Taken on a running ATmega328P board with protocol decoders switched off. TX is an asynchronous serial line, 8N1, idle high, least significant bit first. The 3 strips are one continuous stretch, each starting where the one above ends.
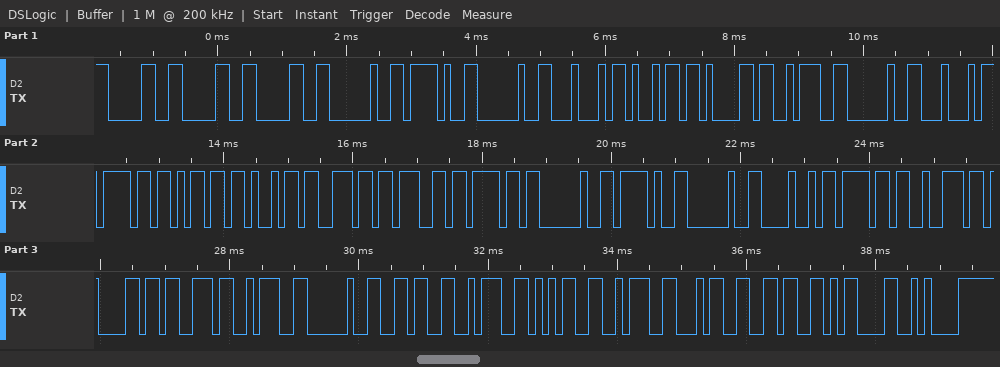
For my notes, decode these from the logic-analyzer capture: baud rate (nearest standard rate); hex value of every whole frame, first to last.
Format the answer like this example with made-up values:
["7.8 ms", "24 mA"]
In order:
["9600 baud", "30 30 30 20 2F 20 44 69 61 3A 20 44 6F 6D 69 6E 67 6F 20 2F 20 48 6F 72 61 73 3A 20 36 3A 35 3A 34 36 0D 0A"]
